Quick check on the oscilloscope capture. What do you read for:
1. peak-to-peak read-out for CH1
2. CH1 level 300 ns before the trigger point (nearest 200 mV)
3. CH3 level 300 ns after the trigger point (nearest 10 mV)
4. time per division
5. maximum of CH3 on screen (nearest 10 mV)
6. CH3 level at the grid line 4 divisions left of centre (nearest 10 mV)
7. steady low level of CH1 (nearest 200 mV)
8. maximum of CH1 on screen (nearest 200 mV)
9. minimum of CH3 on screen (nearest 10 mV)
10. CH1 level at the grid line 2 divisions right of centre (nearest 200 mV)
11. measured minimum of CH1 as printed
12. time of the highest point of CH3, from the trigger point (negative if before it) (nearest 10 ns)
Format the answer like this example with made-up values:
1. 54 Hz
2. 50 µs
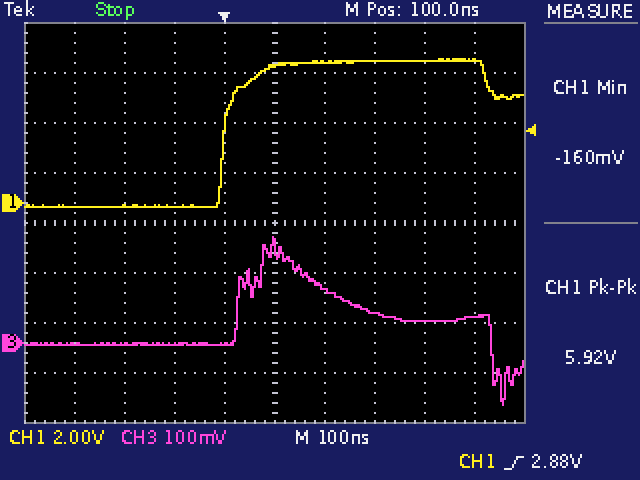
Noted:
1. 5.92 V
2. -200 mV
3. 60 mV
4. 100 ns
5. 210 mV
6. 0 mV
7. -200 mV
8. 5.8 V
9. -120 mV
10. 5.6 V
11. -160 mV
12. +100 ns
